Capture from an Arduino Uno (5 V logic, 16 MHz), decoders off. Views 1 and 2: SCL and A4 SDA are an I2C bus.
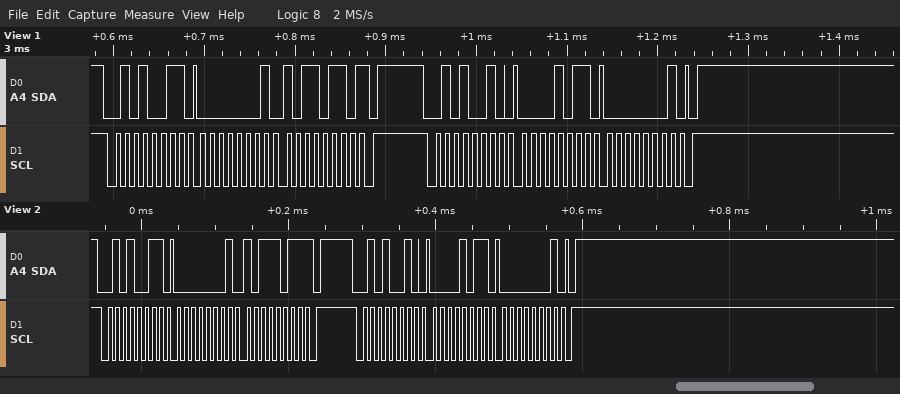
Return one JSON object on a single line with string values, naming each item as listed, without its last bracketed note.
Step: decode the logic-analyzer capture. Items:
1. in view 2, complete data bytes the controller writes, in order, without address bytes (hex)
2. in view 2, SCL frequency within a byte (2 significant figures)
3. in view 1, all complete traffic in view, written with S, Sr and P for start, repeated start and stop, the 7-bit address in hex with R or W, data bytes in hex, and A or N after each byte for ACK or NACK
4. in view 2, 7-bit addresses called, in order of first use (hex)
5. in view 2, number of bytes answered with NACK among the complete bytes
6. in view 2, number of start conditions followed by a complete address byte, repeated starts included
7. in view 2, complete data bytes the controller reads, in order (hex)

{"in view 2, complete data bytes the controller writes, in order, without address bytes": "0B 01", "in view 2, SCL frequency within a byte": "100 kHz", "in view 1, all complete traffic in view, written with S, Sr and P for start, repeated start and stop, the 7-bit address in hex with R or W, data bytes in hex, and A or N after each byte for ACK or NACK": "S 29R A 01 A B6 N P S 29W A 0B A 01 A P", "in view 2, 7-bit addresses called, in order of first use": "0x29", "in view 2, number of bytes answered with NACK among the complete bytes": "1", "in view 2, number of start conditions followed by a complete address byte, repeated starts included": "2", "in view 2, complete data bytes the controller reads, in order": "01 BB"}
